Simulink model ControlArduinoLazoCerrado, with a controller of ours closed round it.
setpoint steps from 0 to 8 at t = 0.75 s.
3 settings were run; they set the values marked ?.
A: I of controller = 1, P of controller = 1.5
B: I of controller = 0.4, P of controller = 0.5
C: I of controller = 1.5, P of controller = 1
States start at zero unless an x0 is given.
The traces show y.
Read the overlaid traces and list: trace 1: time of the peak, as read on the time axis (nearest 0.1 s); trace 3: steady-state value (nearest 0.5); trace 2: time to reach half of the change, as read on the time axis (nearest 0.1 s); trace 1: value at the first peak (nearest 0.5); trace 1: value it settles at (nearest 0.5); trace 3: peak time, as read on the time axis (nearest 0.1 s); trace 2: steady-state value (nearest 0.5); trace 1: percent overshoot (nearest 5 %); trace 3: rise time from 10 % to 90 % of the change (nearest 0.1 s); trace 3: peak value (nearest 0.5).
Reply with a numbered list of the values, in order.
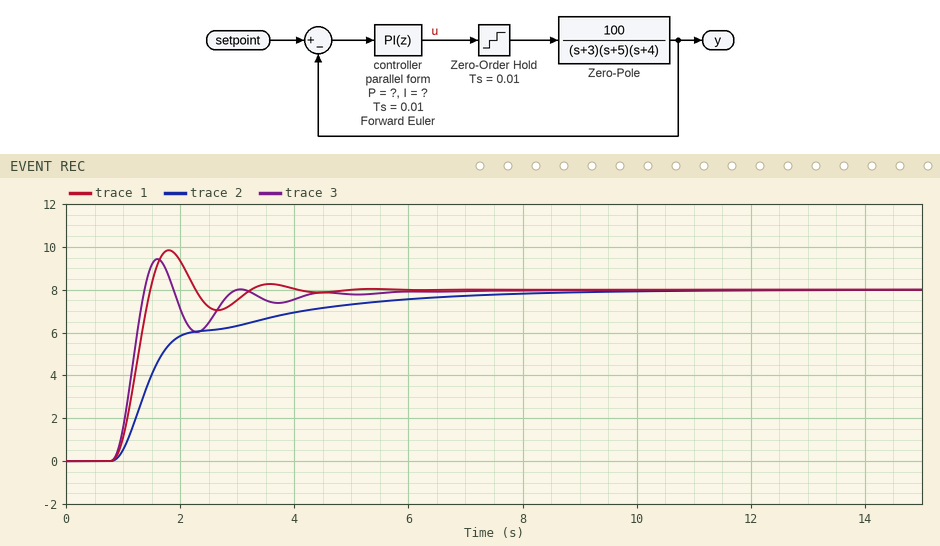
1. 1.8 s
2. 8.0
3. 1.5 s
4. 10.0
5. 8.0
6. 1.6 s
7. 8.0
8. 25 %
9. 0.4 s
10. 9.5
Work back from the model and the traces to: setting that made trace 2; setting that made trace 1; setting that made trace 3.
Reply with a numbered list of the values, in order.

1. B
2. C
3. A
